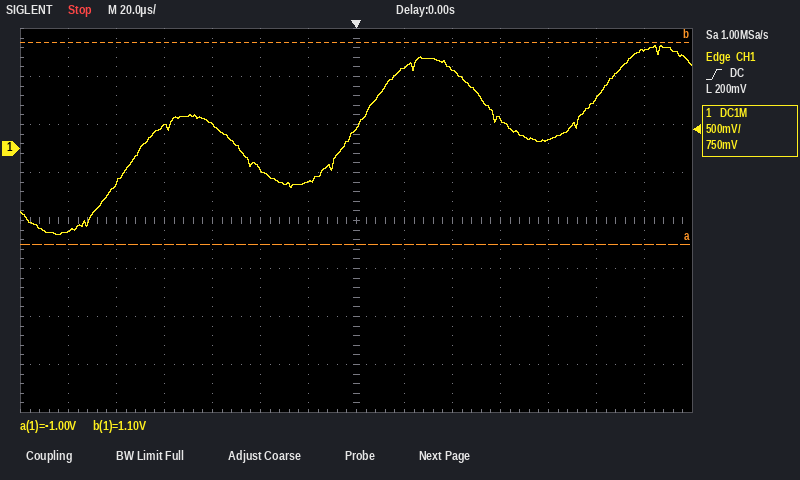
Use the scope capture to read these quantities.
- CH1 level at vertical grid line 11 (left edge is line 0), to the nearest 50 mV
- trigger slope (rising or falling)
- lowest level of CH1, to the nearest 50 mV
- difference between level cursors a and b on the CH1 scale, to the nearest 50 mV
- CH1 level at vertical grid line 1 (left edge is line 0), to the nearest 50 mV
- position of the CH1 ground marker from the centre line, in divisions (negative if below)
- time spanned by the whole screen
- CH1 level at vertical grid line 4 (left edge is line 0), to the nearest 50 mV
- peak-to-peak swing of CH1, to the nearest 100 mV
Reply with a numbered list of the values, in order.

1. 100 mV
2. rising
3. -900 mV
4. 2.10 V
5. -850 mV
6. +1.5 div
7. 280 µs
8. 250 mV
9. 2.00 V
